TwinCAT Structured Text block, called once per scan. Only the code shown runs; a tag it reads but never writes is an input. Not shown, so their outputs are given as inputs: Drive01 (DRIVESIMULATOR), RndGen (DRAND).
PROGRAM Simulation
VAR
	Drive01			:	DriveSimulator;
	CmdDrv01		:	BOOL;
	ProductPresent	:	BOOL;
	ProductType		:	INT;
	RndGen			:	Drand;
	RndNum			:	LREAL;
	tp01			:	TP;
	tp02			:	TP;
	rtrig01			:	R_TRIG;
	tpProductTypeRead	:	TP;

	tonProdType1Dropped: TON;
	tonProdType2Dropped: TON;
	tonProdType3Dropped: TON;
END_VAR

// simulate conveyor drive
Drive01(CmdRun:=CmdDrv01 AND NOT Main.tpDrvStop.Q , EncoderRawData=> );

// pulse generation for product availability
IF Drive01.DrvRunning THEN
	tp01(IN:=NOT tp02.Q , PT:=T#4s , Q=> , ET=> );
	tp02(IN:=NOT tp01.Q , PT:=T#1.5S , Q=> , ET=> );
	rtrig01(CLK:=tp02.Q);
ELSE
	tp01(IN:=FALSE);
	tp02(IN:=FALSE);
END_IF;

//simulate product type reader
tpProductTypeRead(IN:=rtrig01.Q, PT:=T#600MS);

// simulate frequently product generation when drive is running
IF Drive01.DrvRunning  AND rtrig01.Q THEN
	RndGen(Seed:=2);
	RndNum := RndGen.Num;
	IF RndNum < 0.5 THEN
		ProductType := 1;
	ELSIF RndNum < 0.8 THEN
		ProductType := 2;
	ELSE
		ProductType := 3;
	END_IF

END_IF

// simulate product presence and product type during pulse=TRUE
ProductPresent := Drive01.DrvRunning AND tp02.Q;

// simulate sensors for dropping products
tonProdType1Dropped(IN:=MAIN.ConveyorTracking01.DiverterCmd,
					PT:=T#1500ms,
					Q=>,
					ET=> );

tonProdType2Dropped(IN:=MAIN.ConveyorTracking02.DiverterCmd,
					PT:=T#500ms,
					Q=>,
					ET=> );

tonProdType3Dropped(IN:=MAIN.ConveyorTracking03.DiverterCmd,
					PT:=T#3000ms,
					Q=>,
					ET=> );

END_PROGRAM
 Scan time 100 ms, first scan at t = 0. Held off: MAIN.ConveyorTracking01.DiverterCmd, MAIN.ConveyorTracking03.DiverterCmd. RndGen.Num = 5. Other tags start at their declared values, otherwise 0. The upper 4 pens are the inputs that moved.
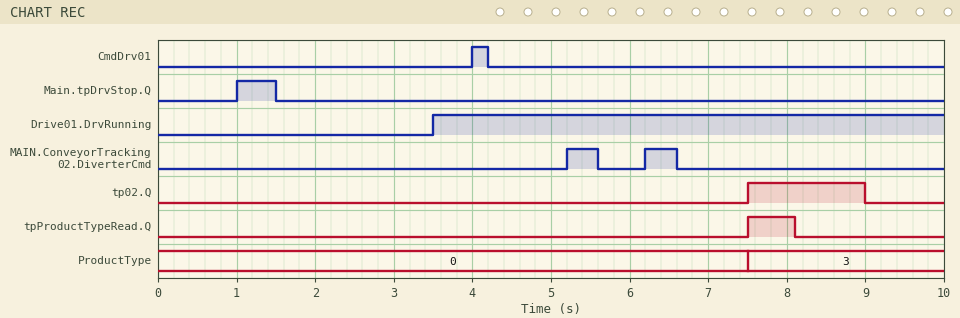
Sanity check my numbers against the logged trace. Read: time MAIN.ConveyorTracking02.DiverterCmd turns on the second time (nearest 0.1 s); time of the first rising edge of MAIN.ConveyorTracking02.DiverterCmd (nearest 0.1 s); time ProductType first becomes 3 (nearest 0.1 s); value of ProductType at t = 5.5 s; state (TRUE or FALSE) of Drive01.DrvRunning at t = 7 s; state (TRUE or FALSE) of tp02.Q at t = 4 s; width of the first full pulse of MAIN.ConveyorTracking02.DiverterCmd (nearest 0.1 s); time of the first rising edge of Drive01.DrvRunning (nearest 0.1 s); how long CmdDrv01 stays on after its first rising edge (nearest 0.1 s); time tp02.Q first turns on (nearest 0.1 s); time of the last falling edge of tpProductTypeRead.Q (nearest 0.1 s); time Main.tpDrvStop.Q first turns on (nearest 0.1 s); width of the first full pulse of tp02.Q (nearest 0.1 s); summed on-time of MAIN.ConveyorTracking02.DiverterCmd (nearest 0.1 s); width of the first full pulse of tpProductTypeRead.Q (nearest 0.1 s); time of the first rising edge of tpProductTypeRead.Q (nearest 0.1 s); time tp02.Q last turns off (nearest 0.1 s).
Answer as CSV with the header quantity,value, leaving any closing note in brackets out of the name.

quantity,value
time MAIN.ConveyorTracking02.DiverterCmd turns on the second time,6.2 s
time of the first rising edge of MAIN.ConveyorTracking02.DiverterCmd,5.2 s
time ProductType first becomes 3,7.5 s
value of ProductType at t = 5.5 s,0
state (TRUE or FALSE) of Drive01.DrvRunning at t = 7 s,TRUE
state (TRUE or FALSE) of tp02.Q at t = 4 s,FALSE
width of the first full pulse of MAIN.ConveyorTracking02.DiverterCmd,0.4 s
time of the first rising edge of Drive01.DrvRunning,3.5 s
how long CmdDrv01 stays on after its first rising edge,0.2 s
time tp02.Q first turns on,7.5 s
time of the last falling edge of tpProductTypeRead.Q,8.1 s
time Main.tpDrvStop.Q first turns on,1.0 s
width of the first full pulse of tp02.Q,1.5 s
summed on-time of MAIN.ConveyorTracking02.DiverterCmd,0.8 s
width of the first full pulse of tpProductTypeRead.Q,0.6 s
time of the first rising edge of tpProductTypeRead.Q,7.5 s
time tp02.Q last turns off,9.0 s
